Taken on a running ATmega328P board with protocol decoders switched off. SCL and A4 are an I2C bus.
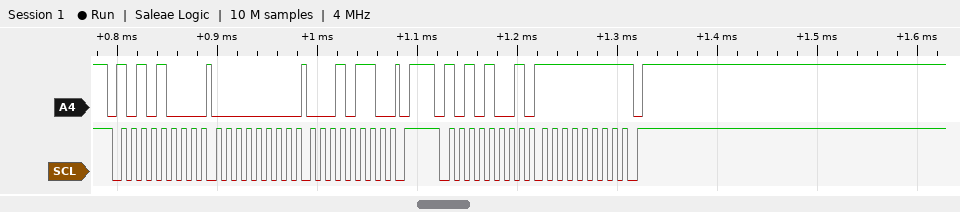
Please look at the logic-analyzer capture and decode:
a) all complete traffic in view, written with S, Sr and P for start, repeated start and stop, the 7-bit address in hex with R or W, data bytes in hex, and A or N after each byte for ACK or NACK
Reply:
S 54W A 00 A 16 A P S 54R A FF N P
